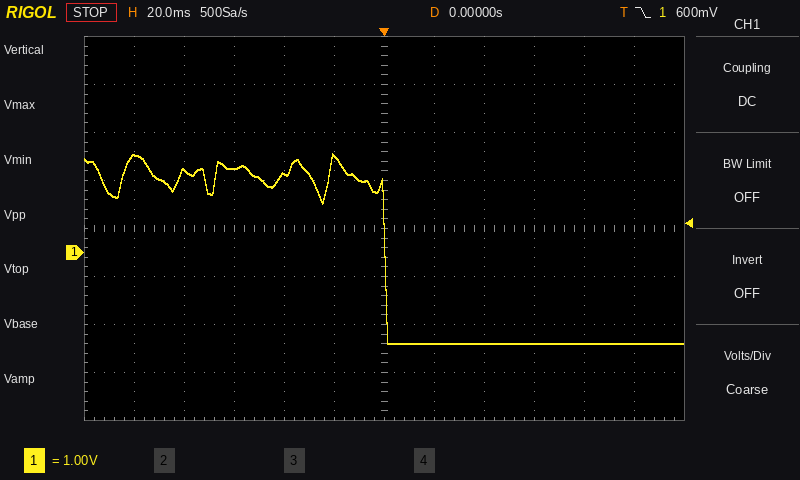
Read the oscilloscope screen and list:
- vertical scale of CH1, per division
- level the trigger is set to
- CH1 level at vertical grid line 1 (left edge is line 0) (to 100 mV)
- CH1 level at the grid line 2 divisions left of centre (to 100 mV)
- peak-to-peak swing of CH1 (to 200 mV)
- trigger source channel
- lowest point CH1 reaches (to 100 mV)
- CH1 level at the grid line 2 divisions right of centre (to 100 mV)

1 V
600 mV
2.0 V
1.6 V
4.0 V
CH1
-1.9 V
-1.9 V
